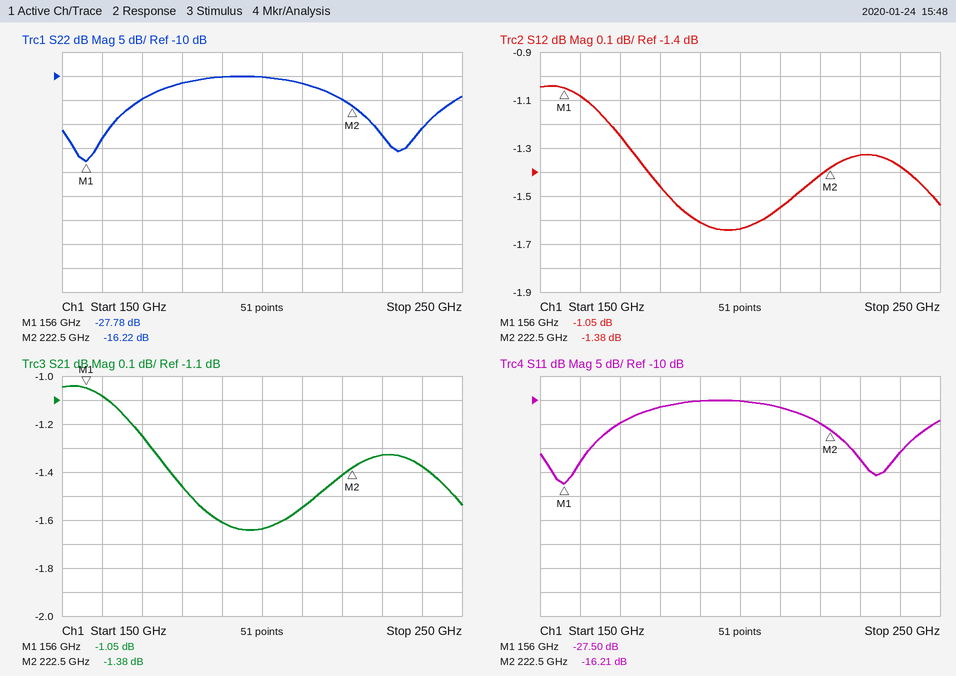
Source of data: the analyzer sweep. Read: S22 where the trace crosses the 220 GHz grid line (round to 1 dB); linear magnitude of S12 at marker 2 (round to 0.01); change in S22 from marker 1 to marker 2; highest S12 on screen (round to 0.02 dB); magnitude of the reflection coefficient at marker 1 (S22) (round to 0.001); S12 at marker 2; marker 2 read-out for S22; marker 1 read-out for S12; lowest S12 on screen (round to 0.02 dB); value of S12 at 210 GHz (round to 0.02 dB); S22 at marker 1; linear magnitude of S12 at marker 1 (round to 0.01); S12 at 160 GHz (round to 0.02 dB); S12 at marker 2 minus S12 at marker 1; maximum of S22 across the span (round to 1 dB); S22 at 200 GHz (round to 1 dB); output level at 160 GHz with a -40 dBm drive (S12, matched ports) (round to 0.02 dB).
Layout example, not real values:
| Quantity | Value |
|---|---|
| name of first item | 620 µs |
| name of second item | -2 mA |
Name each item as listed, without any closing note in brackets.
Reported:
| Quantity | Value |
|---|---|
| S22 where the trace crosses the 220 GHz grid line | -15 dB |
| linear magnitude of S12 at marker 2 | 0.85 |
| change in S22 from marker 1 to marker 2 | 11.56 dB |
| highest S12 on screen | -1.04 dB |
| magnitude of the reflection coefficient at marker 1 (S22) | 0.041 |
| S12 at marker 2 | -1.38 dB |
| marker 2 read-out for S22 | -16.22 dB |
| marker 1 read-out for S12 | -1.05 dB |
| lowest S12 on screen | -1.64 dB |
| value of S12 at 210 GHz | -1.54 dB |
| S22 at marker 1 | -27.78 dB |
| linear magnitude of S12 at marker 1 | 0.89 |
| S12 at 160 GHz | -1.08 dB |
| S12 at marker 2 minus S12 at marker 1 | -0.33 dB |
| maximum of S22 across the span | -10 dB |
| S22 at 200 GHz | -10 dB |
| output level at 160 GHz with a -40 dBm drive (S12, matched ports) | -41.08 dBm |
